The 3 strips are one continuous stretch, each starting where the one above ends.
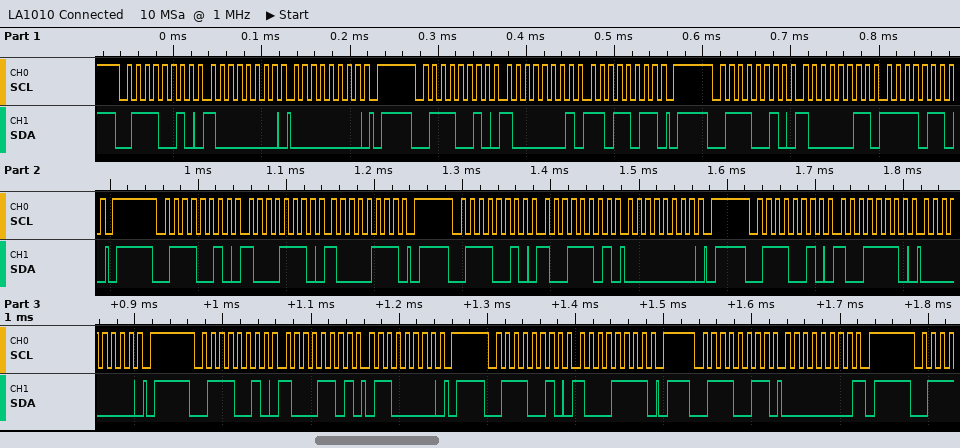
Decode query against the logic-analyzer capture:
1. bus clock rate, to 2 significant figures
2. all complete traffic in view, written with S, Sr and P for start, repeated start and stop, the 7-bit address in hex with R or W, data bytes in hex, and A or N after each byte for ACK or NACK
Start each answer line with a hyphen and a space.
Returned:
- 100 kHz
- S 39W A 80 A 00 A P S 39W A 81 A DB A P S 39W A 83 A F6 A P S 39W A 8E A 87 A P S 39W A 9D A 00 A P S 39W A 9E A 00 A P S 39W A 8D A 60 A P S 39W A 8F A P S 39R A 00 N P
